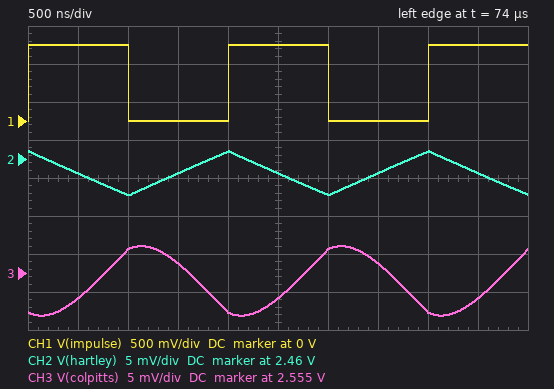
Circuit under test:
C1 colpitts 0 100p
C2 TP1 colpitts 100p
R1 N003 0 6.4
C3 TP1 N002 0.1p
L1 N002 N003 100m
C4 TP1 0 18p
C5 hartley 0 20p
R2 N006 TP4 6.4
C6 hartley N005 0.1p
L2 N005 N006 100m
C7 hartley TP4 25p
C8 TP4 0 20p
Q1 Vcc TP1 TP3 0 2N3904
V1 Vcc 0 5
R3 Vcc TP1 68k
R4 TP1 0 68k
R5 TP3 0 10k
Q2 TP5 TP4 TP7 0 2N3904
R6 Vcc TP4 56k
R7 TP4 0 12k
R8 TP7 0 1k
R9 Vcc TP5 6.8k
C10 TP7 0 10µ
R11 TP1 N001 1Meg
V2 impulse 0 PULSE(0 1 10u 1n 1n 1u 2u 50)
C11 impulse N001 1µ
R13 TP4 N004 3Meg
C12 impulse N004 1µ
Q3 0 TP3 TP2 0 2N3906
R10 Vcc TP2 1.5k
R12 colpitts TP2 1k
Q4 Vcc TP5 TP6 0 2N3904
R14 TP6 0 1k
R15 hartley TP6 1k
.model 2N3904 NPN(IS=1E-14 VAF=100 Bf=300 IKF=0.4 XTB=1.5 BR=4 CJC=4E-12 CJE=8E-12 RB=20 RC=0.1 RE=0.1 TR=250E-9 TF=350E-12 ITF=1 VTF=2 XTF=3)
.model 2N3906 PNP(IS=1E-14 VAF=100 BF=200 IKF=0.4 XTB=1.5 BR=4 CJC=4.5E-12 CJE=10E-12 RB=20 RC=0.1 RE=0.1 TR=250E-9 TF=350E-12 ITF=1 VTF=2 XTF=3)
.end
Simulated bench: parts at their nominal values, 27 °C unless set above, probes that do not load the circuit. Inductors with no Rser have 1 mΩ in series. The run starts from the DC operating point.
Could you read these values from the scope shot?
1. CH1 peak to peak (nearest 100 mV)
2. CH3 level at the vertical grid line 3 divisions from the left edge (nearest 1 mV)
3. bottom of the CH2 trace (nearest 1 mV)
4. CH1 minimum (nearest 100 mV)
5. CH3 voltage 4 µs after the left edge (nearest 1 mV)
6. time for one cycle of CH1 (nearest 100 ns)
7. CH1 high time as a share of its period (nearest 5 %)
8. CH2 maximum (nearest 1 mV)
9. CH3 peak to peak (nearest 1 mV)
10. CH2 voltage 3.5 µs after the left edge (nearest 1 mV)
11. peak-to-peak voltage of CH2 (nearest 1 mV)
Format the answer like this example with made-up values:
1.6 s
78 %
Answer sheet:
1.0 V
2.556 V
2.455 V
0 V
2.550 V
2.0 µs
50 %
2.461 V
9 mV
2.458 V
6 mV
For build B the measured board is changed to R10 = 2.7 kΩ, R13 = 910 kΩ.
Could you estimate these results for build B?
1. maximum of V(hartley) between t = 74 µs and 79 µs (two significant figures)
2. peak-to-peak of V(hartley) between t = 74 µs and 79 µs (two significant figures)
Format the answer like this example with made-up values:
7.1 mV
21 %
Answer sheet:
2.3 V
19 mV
